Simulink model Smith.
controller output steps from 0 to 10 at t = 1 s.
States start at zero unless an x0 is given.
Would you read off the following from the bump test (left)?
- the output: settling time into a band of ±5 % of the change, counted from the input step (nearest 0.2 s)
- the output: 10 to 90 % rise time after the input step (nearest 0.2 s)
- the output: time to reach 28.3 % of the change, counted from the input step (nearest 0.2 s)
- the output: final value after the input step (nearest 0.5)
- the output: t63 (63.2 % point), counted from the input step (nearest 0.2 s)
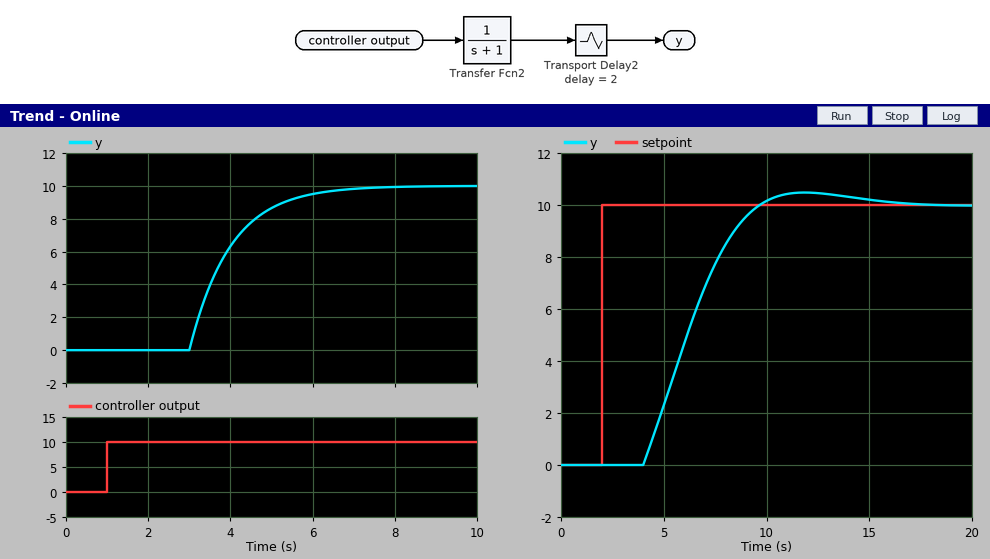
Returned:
5.0 s
2.2 s
2.4 s
10.0
3.0 s
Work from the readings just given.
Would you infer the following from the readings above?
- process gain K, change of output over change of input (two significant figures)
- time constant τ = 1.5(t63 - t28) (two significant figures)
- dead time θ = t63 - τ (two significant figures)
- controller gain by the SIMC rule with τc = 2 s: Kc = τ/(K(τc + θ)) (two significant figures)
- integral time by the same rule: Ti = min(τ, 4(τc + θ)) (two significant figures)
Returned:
1.0
0.90 s
2.1 s
0.22
0.90 s
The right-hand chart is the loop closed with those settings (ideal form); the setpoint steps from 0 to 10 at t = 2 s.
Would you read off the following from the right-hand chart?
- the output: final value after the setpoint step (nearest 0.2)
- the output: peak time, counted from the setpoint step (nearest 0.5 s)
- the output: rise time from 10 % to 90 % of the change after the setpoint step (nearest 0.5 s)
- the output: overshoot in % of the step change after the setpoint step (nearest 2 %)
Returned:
10.0
10.0 s
4.0 s
4 %
